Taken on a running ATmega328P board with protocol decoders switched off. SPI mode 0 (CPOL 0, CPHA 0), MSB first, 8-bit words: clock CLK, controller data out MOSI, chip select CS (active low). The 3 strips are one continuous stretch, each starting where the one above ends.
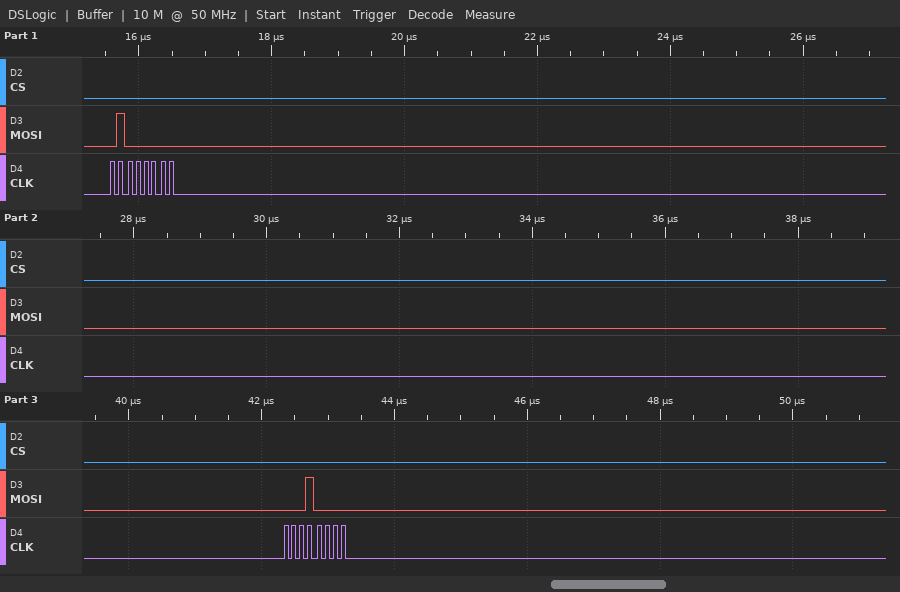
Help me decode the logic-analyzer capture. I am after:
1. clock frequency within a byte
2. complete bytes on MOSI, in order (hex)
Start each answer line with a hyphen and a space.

- 8 MHz
- 40 10
